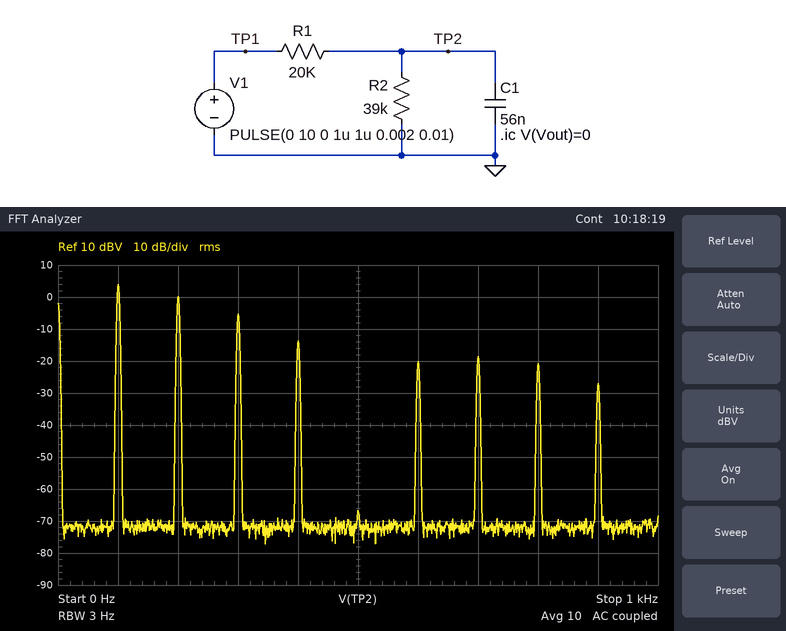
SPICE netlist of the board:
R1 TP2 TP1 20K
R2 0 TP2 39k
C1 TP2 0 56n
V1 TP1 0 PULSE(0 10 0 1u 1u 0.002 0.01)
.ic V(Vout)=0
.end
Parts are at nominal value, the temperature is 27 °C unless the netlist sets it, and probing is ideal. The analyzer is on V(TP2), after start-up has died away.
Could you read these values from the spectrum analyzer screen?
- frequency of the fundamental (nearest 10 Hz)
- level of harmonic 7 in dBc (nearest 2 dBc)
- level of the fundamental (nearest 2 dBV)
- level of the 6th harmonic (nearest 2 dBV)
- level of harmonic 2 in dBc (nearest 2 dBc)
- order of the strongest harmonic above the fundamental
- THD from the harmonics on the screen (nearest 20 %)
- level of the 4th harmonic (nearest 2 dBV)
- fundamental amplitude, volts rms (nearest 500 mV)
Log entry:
100 Hz
-22 dBc
4 dBV
-20 dBV
-4 dBc
2
80 %
-14 dBV
1.5 V
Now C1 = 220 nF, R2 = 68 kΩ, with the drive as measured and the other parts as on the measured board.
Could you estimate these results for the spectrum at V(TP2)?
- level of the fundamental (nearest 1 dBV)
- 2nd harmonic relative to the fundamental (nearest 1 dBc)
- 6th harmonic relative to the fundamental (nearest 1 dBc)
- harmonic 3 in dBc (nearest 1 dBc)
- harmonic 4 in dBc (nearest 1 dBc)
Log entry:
-1 dBV
-7 dBc
-30 dBc
-14 dBc
-23 dBc
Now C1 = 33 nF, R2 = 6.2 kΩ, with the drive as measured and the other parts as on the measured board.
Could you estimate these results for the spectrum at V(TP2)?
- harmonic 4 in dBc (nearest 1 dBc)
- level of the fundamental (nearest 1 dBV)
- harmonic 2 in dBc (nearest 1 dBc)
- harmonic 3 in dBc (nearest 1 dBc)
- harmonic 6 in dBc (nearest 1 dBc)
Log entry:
-13 dBc
-4 dBV
-2 dBc
-6 dBc
-17 dBc
